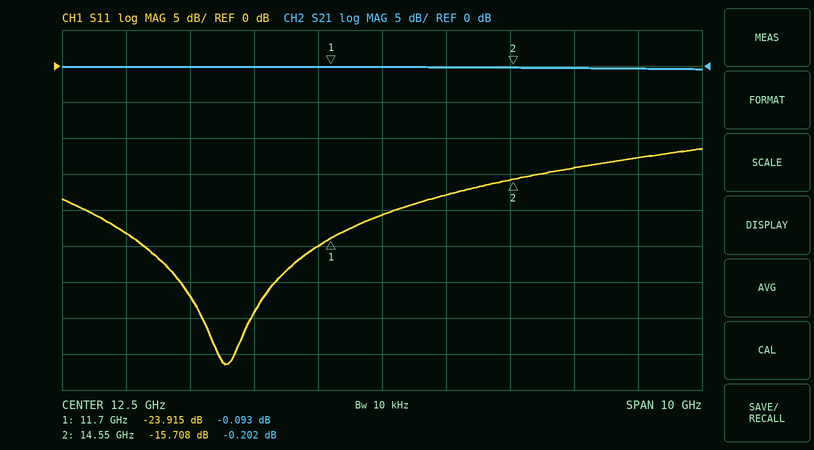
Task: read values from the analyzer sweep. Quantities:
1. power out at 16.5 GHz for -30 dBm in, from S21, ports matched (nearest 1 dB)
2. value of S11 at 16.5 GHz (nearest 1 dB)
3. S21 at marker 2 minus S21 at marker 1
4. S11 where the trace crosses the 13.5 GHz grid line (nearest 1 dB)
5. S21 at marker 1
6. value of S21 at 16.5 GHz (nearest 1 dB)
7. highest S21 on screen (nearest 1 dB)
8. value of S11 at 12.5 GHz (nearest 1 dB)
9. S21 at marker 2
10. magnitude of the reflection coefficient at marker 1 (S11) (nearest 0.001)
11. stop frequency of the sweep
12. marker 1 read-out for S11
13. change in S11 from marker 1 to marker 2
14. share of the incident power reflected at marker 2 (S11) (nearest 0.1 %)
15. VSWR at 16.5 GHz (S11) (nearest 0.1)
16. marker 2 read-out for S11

-30 dBm
-13 dB
-0.109 dB
-18 dB
-0.093 dB
0 dB
0 dB
-21 dB
-0.202 dB
0.064
17.5 GHz
-23.915 dB
8.207 dB
2.7 %
1.6
-15.708 dB
